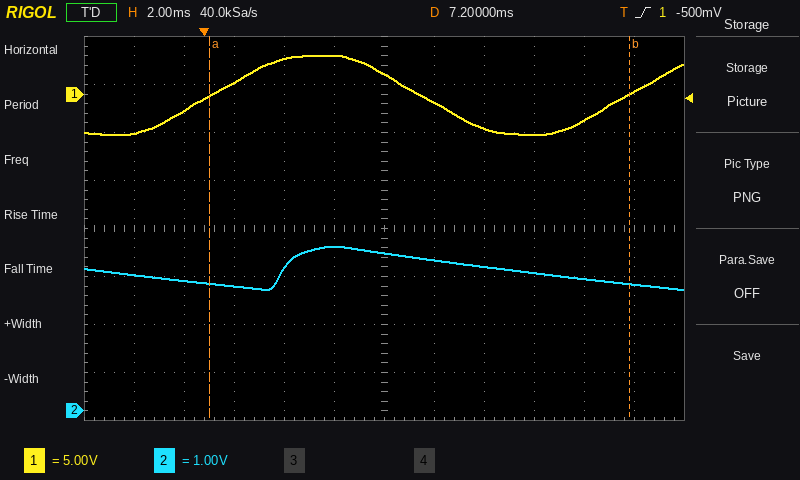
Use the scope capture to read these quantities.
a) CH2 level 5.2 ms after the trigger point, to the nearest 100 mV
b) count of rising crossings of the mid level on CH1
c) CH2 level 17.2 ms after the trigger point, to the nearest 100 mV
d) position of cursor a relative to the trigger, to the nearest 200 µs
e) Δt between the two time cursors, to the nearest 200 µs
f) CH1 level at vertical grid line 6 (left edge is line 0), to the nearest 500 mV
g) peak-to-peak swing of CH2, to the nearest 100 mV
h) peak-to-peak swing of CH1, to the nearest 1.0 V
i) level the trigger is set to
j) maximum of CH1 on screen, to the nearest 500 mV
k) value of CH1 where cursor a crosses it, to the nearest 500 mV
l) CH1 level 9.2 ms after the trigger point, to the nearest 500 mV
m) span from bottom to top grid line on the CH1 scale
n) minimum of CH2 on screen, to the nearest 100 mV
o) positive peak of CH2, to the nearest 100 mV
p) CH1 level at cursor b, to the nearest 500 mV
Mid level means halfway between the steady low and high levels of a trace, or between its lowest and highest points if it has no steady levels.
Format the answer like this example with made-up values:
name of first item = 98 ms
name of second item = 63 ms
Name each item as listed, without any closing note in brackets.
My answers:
CH2 level 5.2 ms after the trigger point, to the nearest 100 mV = 3.4 V
count of rising crossings of the mid level on CH1 = 2
CH2 level 17.2 ms after the trigger point, to the nearest 100 mV = 2.6 V
position of cursor a relative to the trigger, to the nearest 200 µs = +200 µs
Δt between the two time cursors, to the nearest 200 µs = 16.8 ms
CH1 level at vertical grid line 6 (left edge is line 0), to the nearest 500 mV = 2.0 V
peak-to-peak swing of CH2, to the nearest 100 mV = 900 mV
peak-to-peak swing of CH1, to the nearest 1.0 V = 8.0 V
level the trigger is set to = -500 mV
maximum of CH1 on screen, to the nearest 500 mV = 4.0 V
value of CH1 where cursor a crosses it, to the nearest 500 mV = 0.0 V
CH1 level 9.2 ms after the trigger point, to the nearest 500 mV = -1.0 V
span from bottom to top grid line on the CH1 scale = 40 V
minimum of CH2 on screen, to the nearest 100 mV = 2.5 V
positive peak of CH2, to the nearest 100 mV = 3.4 V
CH1 level at cursor b, to the nearest 500 mV = 0.0 V
